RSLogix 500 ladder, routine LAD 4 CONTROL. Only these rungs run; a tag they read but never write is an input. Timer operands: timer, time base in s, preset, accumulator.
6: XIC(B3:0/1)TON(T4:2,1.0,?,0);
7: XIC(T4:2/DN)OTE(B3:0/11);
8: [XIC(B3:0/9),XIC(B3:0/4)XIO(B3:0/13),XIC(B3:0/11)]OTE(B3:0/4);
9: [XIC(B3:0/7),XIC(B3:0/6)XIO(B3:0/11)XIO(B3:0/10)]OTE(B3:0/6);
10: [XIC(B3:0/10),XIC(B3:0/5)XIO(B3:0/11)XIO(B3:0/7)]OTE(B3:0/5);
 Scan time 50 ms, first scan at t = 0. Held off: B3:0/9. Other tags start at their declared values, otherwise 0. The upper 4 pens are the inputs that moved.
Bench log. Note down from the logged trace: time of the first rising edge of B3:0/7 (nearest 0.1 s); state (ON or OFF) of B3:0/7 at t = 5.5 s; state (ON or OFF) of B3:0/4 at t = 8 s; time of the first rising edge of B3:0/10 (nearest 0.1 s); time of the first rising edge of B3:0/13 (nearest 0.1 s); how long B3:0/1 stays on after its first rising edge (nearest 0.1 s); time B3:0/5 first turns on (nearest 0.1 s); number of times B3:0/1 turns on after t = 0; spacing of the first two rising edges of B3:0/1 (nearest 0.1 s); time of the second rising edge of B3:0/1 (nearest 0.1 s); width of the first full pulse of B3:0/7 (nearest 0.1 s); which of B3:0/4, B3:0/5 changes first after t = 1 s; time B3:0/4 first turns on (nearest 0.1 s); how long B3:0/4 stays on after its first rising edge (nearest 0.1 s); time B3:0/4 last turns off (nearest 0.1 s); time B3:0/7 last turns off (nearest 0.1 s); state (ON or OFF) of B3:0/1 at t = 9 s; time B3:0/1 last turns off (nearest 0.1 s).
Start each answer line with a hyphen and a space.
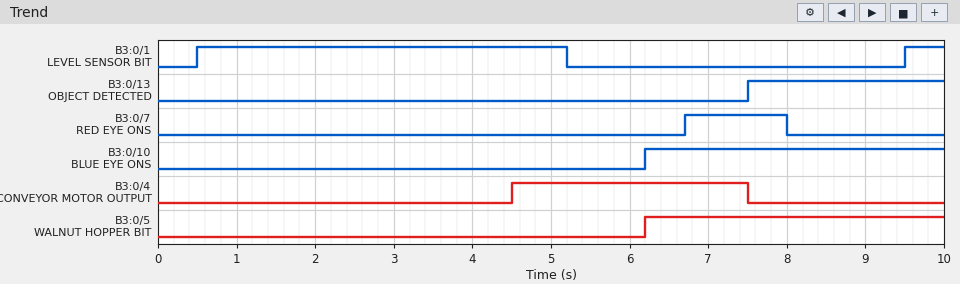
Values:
- 6.7 s
- OFF
- OFF
- 6.2 s
- 7.5 s
- 4.7 s
- 6.2 s
- 2
- 9.0 s
- 9.5 s
- 1.3 s
- B3:0/4
- 4.5 s
- 3.0 s
- 7.5 s
- 8.0 s
- OFF
- 5.2 s
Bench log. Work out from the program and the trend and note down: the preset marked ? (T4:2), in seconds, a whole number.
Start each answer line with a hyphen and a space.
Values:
- 4 s
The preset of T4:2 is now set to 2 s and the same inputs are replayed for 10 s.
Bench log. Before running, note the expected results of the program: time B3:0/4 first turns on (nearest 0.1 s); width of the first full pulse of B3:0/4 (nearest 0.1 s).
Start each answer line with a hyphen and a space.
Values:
- 2.5 s
- 5.0 s
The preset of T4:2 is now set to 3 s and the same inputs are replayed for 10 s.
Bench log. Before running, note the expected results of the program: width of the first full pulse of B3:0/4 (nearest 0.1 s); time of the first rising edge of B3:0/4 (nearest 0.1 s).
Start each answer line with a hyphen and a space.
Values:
- 4.0 s
- 3.5 s
